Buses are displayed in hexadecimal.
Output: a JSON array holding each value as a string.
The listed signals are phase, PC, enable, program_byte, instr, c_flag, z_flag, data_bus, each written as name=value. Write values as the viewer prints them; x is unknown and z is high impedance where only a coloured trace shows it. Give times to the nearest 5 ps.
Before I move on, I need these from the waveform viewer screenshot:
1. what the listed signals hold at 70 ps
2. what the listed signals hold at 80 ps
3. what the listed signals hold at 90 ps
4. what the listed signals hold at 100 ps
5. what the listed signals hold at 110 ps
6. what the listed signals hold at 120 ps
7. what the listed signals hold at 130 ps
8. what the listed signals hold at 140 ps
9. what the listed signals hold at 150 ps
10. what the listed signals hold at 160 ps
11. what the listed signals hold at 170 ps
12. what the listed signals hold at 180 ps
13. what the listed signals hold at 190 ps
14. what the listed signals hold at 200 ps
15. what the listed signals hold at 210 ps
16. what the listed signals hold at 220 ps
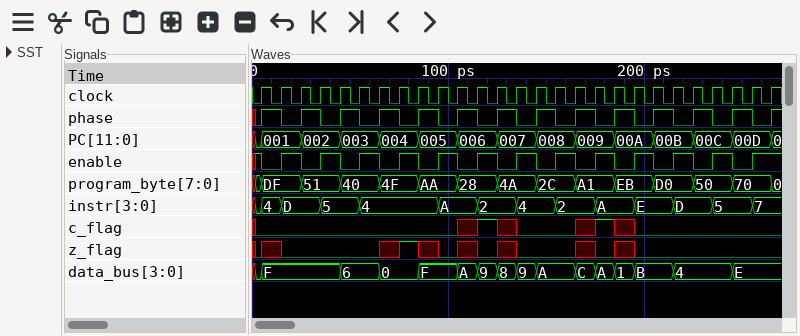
["phase=1, PC=004, enable=0, program_byte=4F, instr=4, c_flag=0, z_flag=x, data_bus=0", "phase=0, PC=004, enable=1, program_byte=4F, instr=4, c_flag=0, z_flag=1, data_bus=0", "phase=1, PC=005, enable=0, program_byte=AA, instr=4, c_flag=0, z_flag=x, data_bus=F", "phase=0, PC=005, enable=1, program_byte=AA, instr=A, c_flag=0, z_flag=0, data_bus=F", "phase=1, PC=006, enable=0, program_byte=28, instr=A, c_flag=x, z_flag=x, data_bus=A", "phase=0, PC=006, enable=1, program_byte=28, instr=2, c_flag=1, z_flag=0, data_bus=9", "phase=1, PC=007, enable=0, program_byte=4A, instr=2, c_flag=x, z_flag=x, data_bus=8", "phase=0, PC=007, enable=1, program_byte=4A, instr=4, c_flag=0, z_flag=0, data_bus=9", "phase=1, PC=008, enable=0, program_byte=2C, instr=4, c_flag=0, z_flag=0, data_bus=A", "phase=0, PC=008, enable=1, program_byte=2C, instr=2, c_flag=0, z_flag=0, data_bus=A", "phase=1, PC=009, enable=0, program_byte=A1, instr=2, c_flag=x, z_flag=x, data_bus=C", "phase=0, PC=009, enable=1, program_byte=A1, instr=A, c_flag=1, z_flag=0, data_bus=A", "phase=1, PC=00A, enable=0, program_byte=EB, instr=A, c_flag=x, z_flag=x, data_bus=1", "phase=0, PC=00A, enable=1, program_byte=EB, instr=E, c_flag=0, z_flag=0, data_bus=B", "phase=1, PC=00B, enable=0, program_byte=D0, instr=E, c_flag=0, z_flag=0, data_bus=B", "phase=0, PC=00B, enable=1, program_byte=D0, instr=D, c_flag=0, z_flag=0, data_bus=4"]
